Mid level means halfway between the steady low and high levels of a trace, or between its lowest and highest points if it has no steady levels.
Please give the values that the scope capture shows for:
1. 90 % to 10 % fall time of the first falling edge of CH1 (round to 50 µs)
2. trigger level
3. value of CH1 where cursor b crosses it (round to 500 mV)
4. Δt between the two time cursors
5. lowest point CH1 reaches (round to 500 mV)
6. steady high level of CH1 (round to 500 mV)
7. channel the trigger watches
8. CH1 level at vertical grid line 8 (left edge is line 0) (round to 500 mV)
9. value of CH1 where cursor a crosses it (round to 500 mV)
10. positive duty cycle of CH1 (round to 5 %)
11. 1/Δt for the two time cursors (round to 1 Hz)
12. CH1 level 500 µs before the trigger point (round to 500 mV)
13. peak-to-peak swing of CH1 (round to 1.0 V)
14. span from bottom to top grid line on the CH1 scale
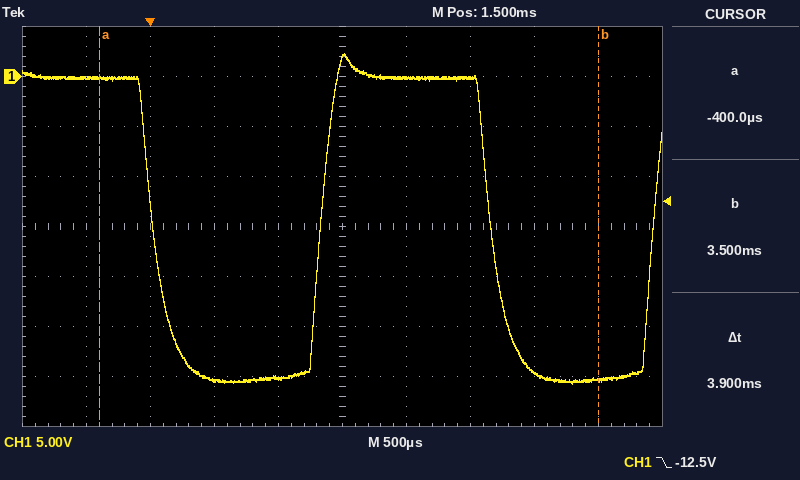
300 µs
-12.5 V
-30.5 V
3.9 ms
-30.5 V
0.0 V
CH1
-29.5 V
0.0 V
50 %
256 Hz
0.0 V
33.0 V
40 V
